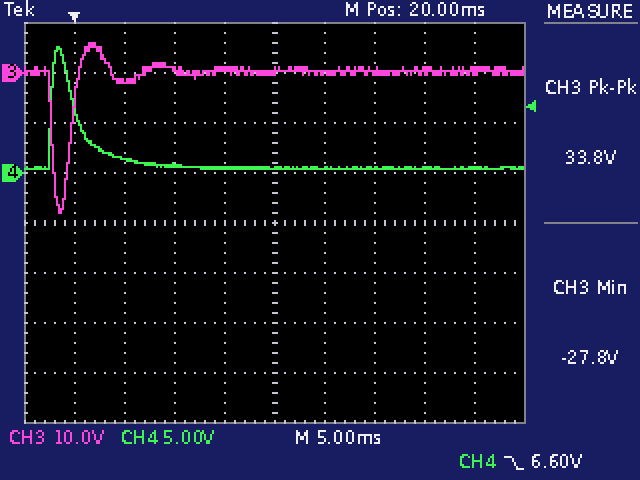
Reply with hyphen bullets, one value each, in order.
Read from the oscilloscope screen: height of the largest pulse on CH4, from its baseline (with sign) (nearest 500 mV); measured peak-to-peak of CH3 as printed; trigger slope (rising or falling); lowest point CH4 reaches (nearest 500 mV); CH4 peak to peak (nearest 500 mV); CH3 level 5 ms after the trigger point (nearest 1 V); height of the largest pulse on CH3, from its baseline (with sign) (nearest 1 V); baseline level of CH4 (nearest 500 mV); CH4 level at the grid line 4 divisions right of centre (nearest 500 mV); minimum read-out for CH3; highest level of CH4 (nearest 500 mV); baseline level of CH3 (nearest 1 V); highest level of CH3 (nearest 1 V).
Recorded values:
- +12.0 V
- 33.8 V
- falling
- 500 mV
- 12.0 V
- -2 V
- -28 V
- 500 mV
- 500 mV
- -27.8 V
- 12.5 V
- 0 V
- 6 V
